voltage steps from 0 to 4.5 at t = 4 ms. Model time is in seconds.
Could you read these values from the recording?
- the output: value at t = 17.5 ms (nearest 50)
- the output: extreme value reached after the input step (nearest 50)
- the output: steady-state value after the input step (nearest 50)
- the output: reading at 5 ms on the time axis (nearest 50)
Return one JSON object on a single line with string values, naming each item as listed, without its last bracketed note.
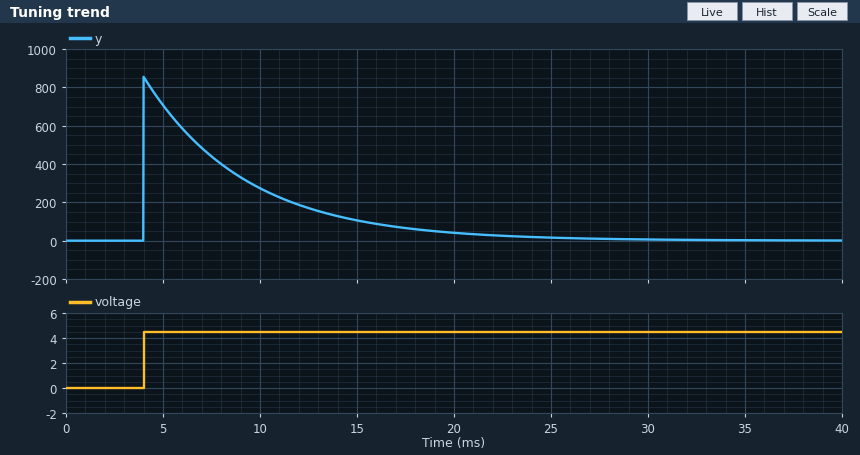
{"the output: value at t = 17.5 ms": "50", "the output: extreme value reached after the input step": "850", "the output: steady-state value after the input step": "0", "the output: reading at 5 ms on the time axis": "700"}
